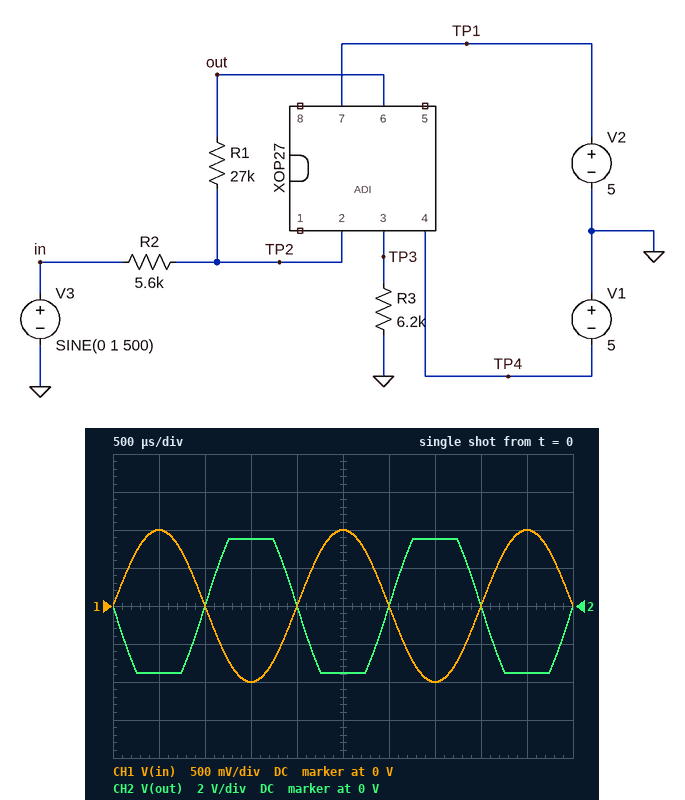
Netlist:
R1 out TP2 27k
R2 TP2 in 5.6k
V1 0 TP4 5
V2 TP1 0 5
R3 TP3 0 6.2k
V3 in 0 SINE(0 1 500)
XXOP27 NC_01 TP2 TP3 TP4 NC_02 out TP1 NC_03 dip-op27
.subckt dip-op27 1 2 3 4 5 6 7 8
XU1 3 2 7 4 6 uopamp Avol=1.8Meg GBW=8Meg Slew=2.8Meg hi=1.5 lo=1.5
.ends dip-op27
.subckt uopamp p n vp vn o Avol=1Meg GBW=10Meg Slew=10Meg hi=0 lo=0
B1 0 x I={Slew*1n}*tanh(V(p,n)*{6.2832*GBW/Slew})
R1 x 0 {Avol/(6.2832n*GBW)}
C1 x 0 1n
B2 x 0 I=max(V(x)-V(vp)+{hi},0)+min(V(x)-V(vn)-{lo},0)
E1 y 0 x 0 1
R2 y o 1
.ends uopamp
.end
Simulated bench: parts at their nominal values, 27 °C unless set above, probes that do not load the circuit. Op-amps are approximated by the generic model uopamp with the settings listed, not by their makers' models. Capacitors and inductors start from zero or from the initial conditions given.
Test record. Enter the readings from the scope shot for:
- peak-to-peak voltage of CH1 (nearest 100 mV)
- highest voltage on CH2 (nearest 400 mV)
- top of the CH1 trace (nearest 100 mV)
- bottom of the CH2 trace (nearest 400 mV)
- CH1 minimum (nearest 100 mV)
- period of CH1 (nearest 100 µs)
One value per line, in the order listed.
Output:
2.0 V
3.6 V
1.0 V
-3.6 V
-1.0 V
2.0 ms
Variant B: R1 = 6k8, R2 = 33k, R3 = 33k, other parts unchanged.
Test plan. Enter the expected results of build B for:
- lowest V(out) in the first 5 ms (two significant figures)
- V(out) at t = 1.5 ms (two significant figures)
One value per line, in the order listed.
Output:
-210 mV
210 mV
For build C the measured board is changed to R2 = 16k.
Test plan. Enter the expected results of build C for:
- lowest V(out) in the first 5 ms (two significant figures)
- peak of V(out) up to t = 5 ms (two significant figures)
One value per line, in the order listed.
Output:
-1.7 V
1.7 V
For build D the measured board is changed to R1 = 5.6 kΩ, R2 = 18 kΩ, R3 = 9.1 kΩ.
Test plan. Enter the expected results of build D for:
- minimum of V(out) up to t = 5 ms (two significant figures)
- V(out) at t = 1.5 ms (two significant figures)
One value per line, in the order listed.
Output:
-310 mV
310 mV
